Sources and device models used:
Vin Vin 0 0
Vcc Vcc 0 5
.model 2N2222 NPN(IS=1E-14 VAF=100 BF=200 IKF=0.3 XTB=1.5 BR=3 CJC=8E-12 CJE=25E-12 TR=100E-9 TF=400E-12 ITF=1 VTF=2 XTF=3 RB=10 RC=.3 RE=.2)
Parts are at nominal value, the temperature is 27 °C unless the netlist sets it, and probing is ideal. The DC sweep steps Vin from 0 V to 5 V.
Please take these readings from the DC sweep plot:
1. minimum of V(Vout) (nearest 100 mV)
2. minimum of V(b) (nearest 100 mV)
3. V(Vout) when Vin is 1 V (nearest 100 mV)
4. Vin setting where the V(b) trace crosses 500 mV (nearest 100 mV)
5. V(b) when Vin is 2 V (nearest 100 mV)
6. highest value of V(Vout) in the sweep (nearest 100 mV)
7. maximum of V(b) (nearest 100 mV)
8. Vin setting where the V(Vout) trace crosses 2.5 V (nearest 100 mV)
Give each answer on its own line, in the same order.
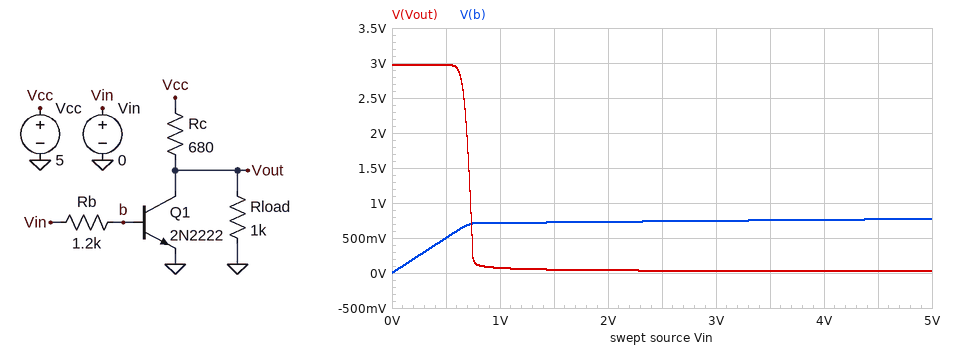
0 V
0 V
100 mV
500 mV
700 mV
3.0 V
800 mV
700 mV
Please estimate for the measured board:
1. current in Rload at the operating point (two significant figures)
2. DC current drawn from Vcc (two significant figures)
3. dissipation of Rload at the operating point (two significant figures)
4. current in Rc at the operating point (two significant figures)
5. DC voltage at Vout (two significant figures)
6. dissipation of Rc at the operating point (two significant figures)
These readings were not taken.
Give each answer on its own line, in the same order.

3.0 mA
3.0 mA
8.9 mW
3.0 mA
3.0 V
6.0 mW
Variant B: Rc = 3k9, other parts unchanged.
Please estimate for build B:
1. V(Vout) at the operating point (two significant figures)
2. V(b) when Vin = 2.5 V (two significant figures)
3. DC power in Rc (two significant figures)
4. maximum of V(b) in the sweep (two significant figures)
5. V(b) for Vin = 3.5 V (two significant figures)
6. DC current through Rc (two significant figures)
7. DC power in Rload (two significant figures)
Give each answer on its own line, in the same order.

1.0 V
720 mV
4.1 mW
760 mV
740 mV
1.0 mA
1.0 mW
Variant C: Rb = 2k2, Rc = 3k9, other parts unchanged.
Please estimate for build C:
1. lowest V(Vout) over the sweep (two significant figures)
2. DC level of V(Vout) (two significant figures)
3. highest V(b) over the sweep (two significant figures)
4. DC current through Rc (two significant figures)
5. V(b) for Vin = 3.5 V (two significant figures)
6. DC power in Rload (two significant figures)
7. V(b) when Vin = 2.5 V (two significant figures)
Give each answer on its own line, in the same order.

13 mV
1.0 V
730 mV
1.0 mA
720 mV
1.0 mW
700 mV
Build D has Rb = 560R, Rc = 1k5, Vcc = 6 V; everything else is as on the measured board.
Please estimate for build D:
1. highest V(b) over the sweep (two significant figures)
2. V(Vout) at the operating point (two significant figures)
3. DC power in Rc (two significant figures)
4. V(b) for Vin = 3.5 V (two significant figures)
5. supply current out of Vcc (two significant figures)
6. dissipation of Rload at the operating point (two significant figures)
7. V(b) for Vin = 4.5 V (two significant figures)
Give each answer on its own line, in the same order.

820 mV
2.4 V
8.6 mW
790 mV
2.4 mA
5.8 mW
810 mV
